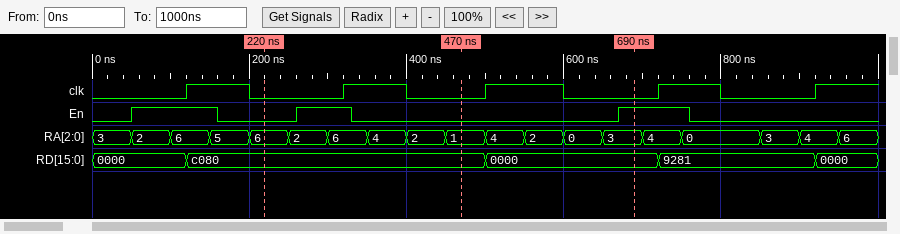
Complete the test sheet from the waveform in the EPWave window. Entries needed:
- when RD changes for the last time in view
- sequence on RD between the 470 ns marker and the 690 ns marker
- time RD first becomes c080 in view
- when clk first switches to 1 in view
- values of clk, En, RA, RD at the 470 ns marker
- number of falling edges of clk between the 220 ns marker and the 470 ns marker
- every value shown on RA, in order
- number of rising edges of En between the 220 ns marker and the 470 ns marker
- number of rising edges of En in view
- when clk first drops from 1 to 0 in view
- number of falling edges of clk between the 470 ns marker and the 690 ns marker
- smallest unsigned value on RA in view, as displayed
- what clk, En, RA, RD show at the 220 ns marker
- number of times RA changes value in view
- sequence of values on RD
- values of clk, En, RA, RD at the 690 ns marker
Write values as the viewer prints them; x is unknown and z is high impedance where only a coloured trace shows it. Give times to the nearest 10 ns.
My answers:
920 ns
c080, 0000
120 ns
120 ns
clk=0, En=0, RA=1, RD=c080
1
3, 2, 6, 5, 6, 2, 6, 4, 2, 1, 4, 2, 0, 3, 4, 0, 3, 4, 6
1
3
200 ns
1
0
clk=0, En=0, RA=6, RD=c080
18
0000, c080, 0000, 9281, 0000
clk=0, En=1, RA=3, RD=0000
